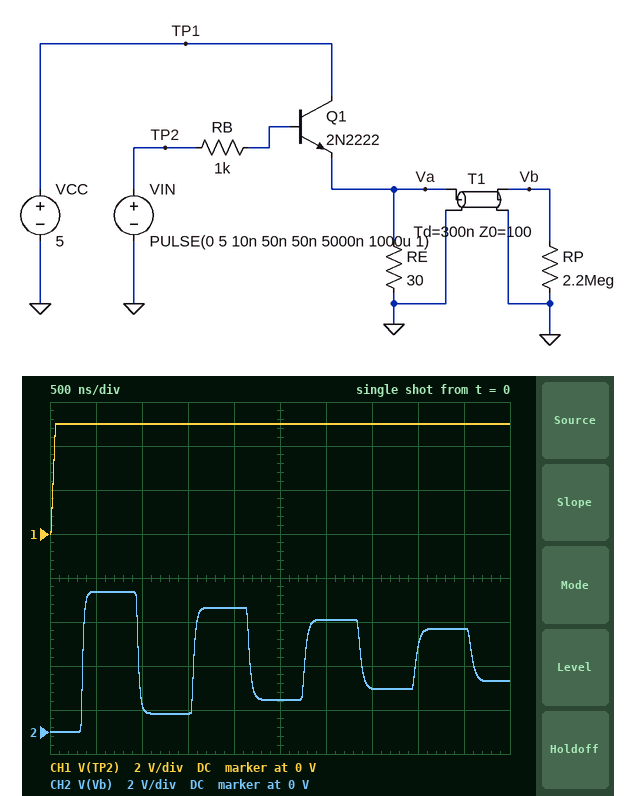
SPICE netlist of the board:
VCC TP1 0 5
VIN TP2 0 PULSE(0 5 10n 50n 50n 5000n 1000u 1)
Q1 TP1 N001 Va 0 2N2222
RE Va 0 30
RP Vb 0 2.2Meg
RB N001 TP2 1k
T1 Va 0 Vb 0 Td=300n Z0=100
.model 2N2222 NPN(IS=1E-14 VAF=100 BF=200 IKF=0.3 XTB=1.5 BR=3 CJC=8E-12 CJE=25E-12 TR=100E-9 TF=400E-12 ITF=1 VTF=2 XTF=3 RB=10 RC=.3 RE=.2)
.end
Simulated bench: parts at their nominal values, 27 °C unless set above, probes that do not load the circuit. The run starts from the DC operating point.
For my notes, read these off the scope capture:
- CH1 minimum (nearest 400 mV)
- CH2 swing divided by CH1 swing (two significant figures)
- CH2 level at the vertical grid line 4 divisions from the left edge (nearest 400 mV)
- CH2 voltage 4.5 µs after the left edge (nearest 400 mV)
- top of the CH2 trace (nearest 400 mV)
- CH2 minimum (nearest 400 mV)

0 V
1.3
5.6 V
4.8 V
6.4 V
0 V
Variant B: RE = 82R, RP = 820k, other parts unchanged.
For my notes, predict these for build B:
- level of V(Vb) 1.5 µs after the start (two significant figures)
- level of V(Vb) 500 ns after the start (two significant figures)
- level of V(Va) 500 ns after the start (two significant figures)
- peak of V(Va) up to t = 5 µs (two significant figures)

950 mV
7.4 V
3.7 V
4.5 V
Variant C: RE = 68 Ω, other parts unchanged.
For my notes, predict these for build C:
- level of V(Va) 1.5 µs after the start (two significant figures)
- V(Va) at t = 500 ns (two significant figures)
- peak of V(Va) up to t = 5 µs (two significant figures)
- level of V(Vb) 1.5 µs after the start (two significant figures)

3.7 V
3.6 V
4.4 V
940 mV
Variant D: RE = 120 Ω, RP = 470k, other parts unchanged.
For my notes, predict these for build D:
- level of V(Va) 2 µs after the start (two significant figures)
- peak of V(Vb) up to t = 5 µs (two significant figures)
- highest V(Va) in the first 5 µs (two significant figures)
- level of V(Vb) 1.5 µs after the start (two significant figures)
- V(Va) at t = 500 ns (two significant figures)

4.2 V
7.6 V
4.7 V
1.0 V
3.8 V
